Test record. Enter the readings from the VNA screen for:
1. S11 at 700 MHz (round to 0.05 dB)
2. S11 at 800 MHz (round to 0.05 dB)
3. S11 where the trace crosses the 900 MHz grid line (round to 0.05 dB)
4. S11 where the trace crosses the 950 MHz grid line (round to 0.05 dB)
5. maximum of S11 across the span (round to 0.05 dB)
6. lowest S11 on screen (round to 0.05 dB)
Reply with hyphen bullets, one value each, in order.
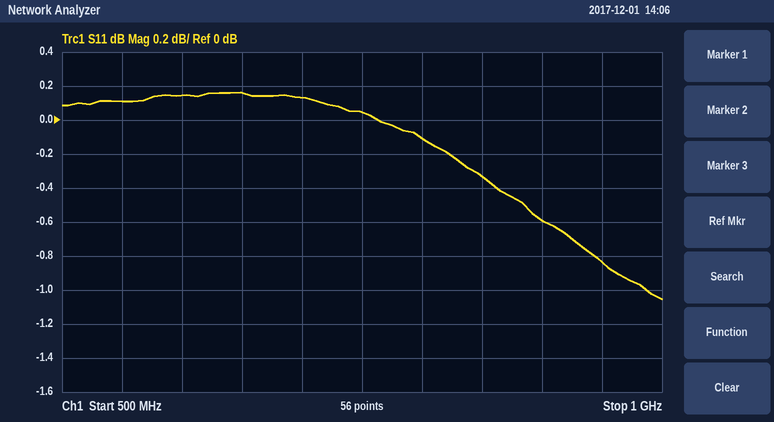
- 0.15 dB
- -0.10 dB
- -0.60 dB
- -0.85 dB
- 0.15 dB
- -1.05 dB
